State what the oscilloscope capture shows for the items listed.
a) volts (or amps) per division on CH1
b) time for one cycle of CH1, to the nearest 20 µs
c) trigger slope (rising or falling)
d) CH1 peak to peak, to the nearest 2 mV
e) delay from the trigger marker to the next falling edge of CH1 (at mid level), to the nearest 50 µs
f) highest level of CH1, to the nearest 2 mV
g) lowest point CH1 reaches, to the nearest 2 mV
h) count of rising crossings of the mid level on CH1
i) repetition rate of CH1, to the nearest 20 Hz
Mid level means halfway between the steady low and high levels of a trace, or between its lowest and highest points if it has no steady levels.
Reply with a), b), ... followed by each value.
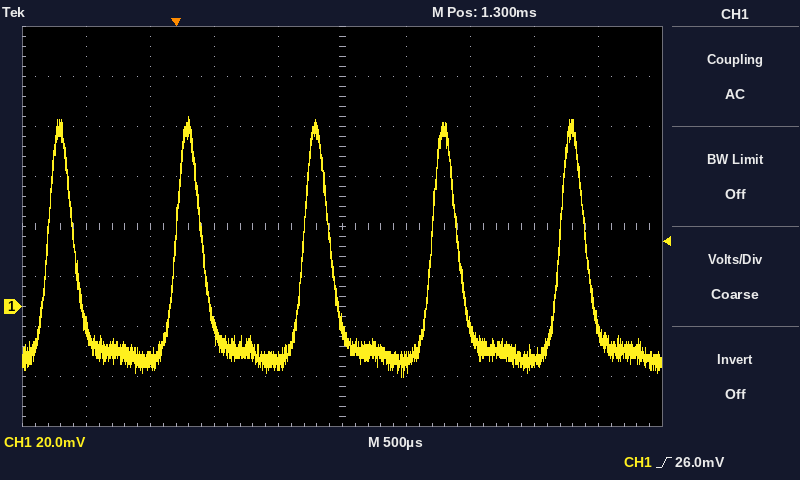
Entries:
a) 20 mV
b) 1.00 ms
c) rising
d) 104 mV
e) 200 µs
f) 76 mV
g) -28 mV
h) 5
i) 1.00 kHz
